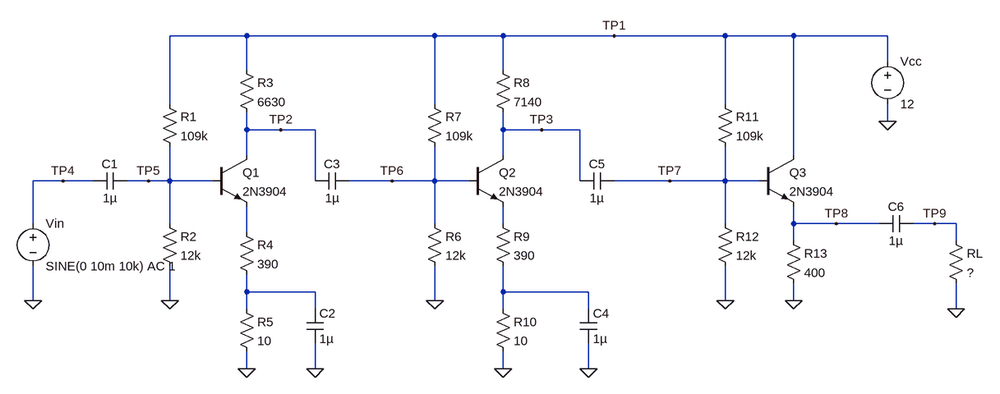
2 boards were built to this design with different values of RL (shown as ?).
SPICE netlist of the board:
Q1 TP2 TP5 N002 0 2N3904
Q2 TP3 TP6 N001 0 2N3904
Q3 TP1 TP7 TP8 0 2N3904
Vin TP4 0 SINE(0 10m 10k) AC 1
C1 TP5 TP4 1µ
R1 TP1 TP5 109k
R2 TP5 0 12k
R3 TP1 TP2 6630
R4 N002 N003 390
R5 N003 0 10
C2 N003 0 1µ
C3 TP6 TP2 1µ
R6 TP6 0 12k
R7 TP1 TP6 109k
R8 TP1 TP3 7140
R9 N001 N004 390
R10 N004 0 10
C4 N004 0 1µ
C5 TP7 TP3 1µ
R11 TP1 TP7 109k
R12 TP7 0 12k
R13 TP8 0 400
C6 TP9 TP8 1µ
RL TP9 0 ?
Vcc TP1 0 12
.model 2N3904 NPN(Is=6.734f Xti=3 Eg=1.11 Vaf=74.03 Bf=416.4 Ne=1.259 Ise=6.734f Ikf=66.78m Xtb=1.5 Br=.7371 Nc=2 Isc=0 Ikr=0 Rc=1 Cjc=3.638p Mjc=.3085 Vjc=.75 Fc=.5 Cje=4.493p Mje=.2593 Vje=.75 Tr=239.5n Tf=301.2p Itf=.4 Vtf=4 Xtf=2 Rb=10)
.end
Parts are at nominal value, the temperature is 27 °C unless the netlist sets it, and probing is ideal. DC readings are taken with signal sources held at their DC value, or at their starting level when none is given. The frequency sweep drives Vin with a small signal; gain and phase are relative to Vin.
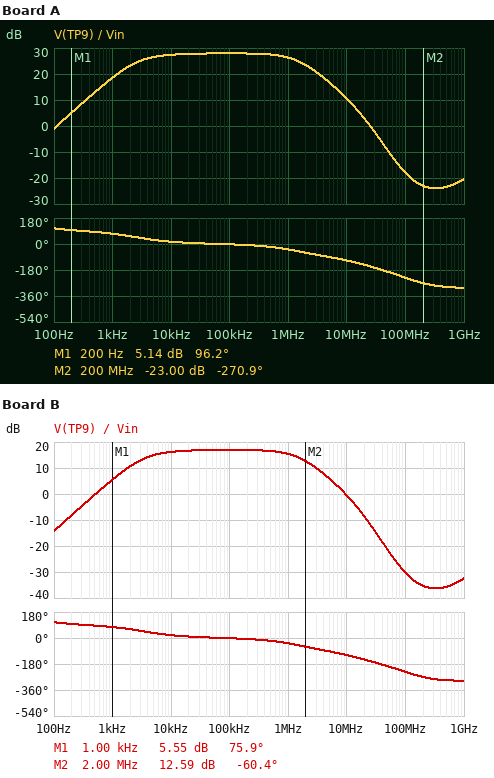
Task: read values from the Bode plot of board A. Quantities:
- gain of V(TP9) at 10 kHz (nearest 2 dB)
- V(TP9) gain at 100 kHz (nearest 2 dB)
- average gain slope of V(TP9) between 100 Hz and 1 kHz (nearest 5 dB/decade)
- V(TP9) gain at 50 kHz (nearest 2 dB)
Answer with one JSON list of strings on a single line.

["28 dB", "28 dB", "20 dB/decade", "28 dB"]
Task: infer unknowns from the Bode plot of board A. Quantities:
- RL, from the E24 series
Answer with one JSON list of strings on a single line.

["18 Ω"]
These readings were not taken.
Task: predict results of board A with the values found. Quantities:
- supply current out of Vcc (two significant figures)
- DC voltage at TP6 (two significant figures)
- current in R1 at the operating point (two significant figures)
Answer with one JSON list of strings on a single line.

["3.6 mA", "1.1 V", "100 µA"]
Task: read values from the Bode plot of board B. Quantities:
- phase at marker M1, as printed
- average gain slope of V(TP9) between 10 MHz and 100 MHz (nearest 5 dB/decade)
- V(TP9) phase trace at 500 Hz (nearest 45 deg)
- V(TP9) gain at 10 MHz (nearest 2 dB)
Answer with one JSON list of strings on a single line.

["75.9 deg", "-30 dB/decade", "90 deg", "0 dB"]
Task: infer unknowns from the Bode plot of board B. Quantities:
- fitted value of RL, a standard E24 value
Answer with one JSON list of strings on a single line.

["3.9 Ω"]
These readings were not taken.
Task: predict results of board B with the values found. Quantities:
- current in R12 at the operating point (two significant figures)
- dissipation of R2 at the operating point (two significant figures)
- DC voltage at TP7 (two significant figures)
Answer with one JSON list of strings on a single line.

["93 µA", "100 µW", "1.1 V"]
